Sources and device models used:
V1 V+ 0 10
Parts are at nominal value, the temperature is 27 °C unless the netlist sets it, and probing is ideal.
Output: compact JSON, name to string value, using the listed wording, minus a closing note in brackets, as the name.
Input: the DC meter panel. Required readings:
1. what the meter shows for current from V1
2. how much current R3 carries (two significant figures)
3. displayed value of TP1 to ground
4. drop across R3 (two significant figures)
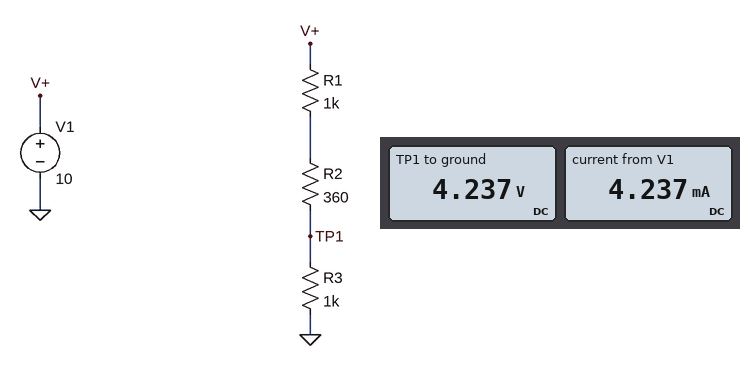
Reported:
{"what the meter shows for current from V1": "4.237 mA", "how much current R3 carries": "4.2 mA", "displayed value of TP1 to ground": "4.237 V", "drop across R3": "4.2 V"}
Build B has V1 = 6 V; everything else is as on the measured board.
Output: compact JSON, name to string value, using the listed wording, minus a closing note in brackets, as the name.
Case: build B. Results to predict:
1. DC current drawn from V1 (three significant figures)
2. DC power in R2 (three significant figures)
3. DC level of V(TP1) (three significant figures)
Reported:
{"DC current drawn from V1": "2.54 mA", "DC power in R2": "2.33 mW", "DC level of V(TP1)": "2.54 V"}
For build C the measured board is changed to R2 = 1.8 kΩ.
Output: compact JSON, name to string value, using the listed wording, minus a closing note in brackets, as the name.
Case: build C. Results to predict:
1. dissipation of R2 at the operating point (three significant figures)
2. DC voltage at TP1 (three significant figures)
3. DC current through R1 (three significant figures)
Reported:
{"dissipation of R2 at the operating point": "12.5 mW", "DC voltage at TP1": "2.63 V", "DC current through R1": "2.63 mA"}
